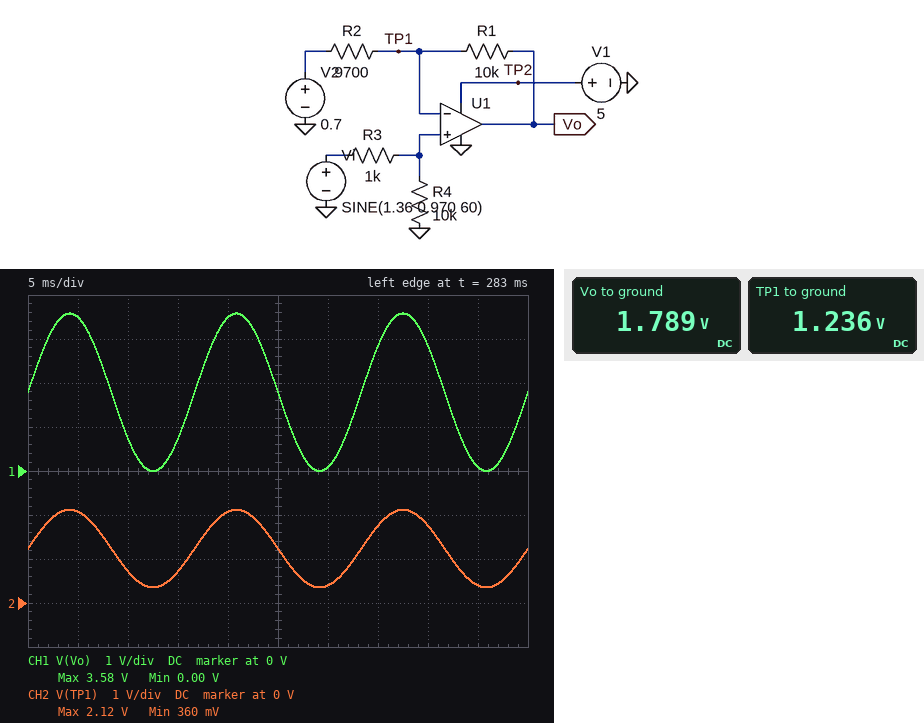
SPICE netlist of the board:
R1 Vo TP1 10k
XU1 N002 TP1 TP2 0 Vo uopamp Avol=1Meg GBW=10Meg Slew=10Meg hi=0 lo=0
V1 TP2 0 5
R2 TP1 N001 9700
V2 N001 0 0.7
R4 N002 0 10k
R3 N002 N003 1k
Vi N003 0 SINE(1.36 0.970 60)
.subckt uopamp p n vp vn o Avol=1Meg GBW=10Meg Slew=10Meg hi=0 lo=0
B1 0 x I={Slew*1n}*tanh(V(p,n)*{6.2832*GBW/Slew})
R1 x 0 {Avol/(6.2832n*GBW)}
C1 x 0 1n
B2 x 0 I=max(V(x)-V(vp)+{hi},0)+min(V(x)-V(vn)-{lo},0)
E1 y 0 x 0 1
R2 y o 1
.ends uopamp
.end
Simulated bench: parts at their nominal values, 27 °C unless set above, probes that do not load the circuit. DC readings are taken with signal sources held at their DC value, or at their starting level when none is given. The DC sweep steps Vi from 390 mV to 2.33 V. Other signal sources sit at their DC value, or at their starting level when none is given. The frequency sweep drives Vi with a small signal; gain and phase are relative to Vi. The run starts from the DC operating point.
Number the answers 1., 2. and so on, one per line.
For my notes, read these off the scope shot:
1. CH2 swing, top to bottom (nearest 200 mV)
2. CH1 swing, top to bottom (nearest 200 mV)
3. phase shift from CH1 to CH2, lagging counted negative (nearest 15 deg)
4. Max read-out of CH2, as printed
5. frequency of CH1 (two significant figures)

1. 1.8 V
2. 3.6 V
3. 0 deg
4. 2.12 V
5. 60 Hz
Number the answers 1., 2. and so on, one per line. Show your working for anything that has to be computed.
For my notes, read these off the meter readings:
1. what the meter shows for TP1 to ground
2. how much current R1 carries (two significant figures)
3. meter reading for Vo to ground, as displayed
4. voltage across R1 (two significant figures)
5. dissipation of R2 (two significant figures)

1. 1.236 V
2. (1.789 V - 1.236 V) / 10 kΩ = 55 µA
3. 1.789 V
4. 1.789 V - 1.236 V = 550 mV
5. (1.236 V - 700 mV)^2 / 9.7 kΩ = 30 µW
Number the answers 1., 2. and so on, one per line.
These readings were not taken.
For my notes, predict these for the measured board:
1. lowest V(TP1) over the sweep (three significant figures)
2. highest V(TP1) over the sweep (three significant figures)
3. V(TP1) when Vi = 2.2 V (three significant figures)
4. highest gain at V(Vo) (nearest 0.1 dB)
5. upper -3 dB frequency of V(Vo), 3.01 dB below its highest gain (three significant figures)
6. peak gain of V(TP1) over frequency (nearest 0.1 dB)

1. 355 mV
2. 2.12 V
3. 2.00 V
4. 5.3 dB
5. 4.92 MHz
6. -0.8 dB
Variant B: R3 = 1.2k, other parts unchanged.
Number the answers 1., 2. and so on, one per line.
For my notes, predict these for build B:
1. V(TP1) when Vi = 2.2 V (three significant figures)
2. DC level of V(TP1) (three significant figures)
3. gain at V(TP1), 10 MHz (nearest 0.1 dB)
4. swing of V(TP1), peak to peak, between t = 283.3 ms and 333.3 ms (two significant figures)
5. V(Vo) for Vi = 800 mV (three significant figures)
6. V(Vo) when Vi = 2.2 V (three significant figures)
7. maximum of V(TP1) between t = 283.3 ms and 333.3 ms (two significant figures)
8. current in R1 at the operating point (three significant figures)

1. 1.96 V
2. 1.21 V
3. -8.1 dB
4. 1.7 V
5. 729 mV
6. 3.27 V
7. 2.1 V
8. 53.0 µA
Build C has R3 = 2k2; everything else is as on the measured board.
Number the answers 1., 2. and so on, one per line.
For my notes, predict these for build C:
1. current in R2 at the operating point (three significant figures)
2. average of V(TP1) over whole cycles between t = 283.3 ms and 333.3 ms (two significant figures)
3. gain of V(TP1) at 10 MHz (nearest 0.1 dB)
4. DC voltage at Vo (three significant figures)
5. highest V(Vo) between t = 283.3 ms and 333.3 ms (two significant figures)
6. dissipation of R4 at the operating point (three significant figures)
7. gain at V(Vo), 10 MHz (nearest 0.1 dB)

1. 42.8 µA
2. 1.1 V
3. -8.8 dB
4. 1.54 V
5. 3.2 V
6. 124 µW
7. -2.7 dB
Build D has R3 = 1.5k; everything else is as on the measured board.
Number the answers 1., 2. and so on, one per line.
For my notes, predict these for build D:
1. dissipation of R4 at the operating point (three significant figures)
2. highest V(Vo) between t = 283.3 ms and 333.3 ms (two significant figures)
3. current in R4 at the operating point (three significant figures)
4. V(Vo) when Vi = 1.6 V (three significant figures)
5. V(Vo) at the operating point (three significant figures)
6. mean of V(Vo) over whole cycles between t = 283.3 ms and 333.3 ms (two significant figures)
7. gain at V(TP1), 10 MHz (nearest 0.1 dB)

1. 140 µW
2. 3.4 V
3. 118 µA
4. 2.10 V
5. 1.68 V
6. 1.7 V
7. -8.3 dB
